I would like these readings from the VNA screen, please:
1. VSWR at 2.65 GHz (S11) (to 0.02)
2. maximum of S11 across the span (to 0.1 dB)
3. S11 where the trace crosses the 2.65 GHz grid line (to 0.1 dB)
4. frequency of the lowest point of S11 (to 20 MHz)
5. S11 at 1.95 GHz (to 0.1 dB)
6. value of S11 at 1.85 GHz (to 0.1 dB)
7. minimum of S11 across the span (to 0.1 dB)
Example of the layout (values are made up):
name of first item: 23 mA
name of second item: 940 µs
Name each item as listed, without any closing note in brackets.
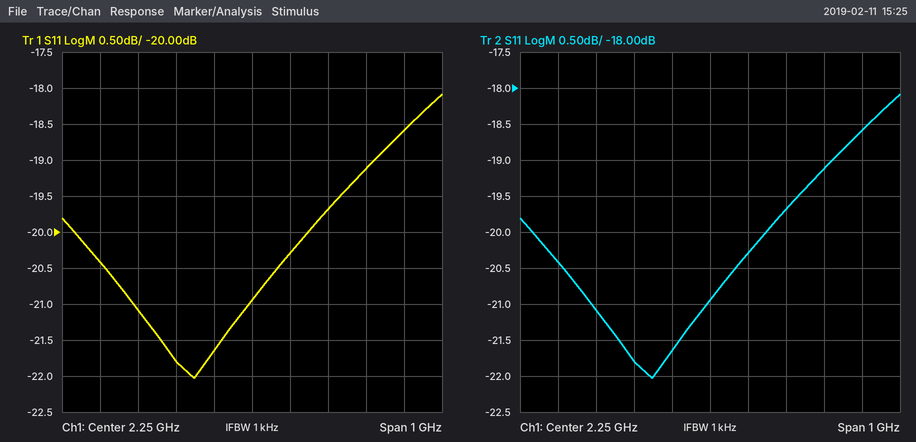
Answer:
VSWR at 2.65 GHz (S11): 1.26
maximum of S11 across the span: -18.1 dB
S11 where the trace crosses the 2.65 GHz grid line: -18.6 dB
frequency of the lowest point of S11: 2.10 GHz
S11 at 1.95 GHz: -21.1 dB
value of S11 at 1.85 GHz: -20.4 dB
minimum of S11 across the span: -22.0 dB
